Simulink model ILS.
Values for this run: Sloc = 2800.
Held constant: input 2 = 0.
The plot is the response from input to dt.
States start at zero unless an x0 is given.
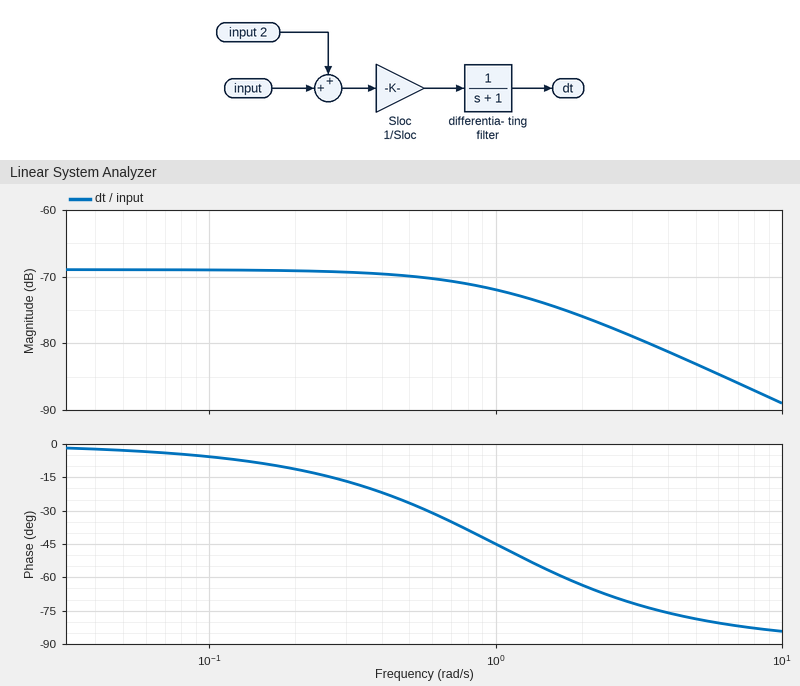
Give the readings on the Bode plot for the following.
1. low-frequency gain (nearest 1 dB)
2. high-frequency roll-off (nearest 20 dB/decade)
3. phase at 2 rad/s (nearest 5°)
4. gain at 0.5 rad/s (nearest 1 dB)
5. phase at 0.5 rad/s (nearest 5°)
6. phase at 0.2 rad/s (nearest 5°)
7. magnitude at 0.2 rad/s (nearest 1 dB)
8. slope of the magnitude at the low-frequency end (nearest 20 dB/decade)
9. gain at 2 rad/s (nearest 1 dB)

-69 dB
-20 dB/decade
-65°
-70 dB
-25°
-10°
-69 dB
0 dB/decade
-76 dB
